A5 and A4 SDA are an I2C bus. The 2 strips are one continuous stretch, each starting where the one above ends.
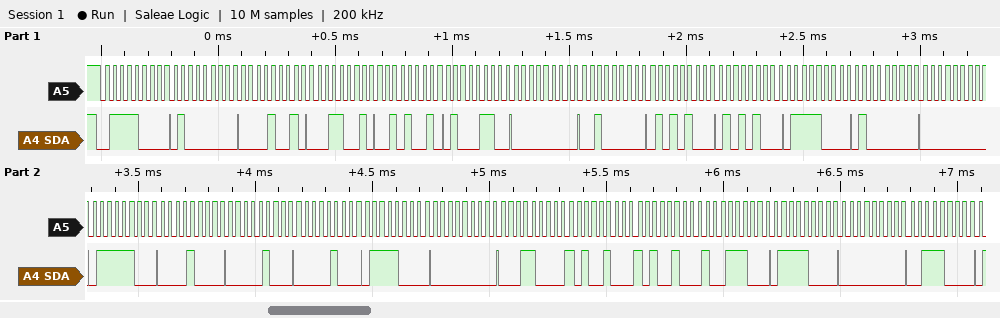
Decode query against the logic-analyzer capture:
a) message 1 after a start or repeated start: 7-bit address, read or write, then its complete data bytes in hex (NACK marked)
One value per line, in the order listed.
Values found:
0x3C write: 40 09 19 29 46 00 20 54 54 78 40 00 7C 08 04 04 78 00 18 A4 A4 9C 78 00 38
